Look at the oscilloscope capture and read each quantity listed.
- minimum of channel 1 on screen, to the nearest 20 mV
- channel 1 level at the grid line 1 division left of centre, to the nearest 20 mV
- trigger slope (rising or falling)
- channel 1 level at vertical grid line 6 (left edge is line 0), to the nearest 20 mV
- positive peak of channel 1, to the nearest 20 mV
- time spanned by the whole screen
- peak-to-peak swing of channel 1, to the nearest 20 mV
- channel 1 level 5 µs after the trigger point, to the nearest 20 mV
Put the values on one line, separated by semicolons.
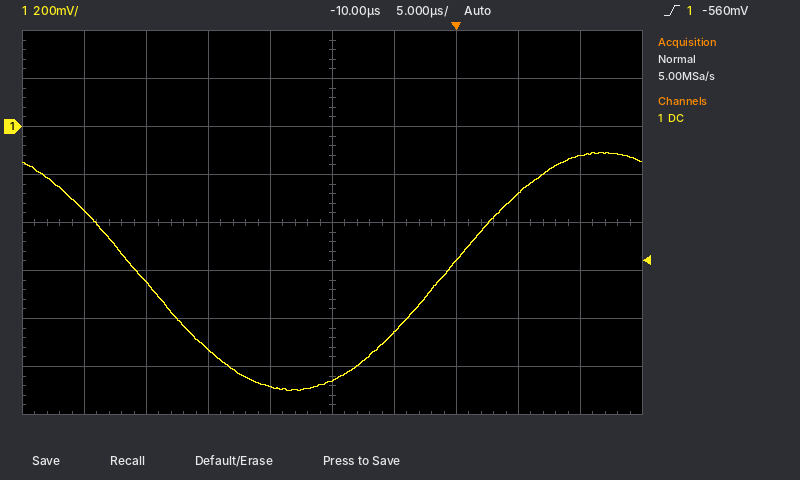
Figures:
-1.10 V; -1.08 V; rising; -860 mV; -100 mV; 50 µs; 1.00 V; -280 mV
